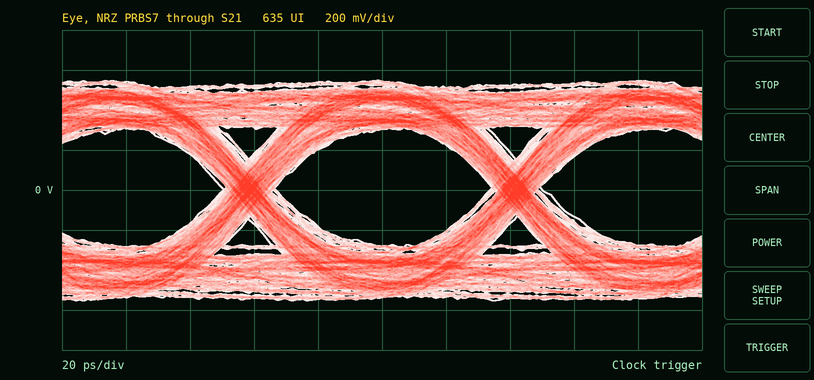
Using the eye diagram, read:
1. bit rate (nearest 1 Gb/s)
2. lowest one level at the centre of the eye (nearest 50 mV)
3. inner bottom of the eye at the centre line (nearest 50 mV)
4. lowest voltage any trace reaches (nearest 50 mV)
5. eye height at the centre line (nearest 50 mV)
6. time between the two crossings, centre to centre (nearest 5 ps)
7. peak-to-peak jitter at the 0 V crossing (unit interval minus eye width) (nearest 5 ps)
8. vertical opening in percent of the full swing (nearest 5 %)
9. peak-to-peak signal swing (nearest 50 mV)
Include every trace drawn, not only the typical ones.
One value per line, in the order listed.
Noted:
12 Gb/s
300 mV
-300 mV
-550 mV
600 mV
85 ps
15 ps
55 %
1.10 V
